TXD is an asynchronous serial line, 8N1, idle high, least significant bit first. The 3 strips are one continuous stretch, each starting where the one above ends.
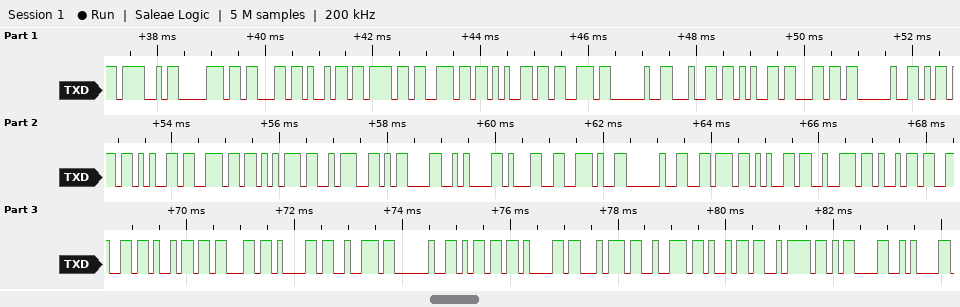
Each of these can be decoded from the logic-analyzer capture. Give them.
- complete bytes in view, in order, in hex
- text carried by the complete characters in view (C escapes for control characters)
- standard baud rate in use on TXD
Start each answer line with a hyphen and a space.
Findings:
- 4F 70 63 69 6F 6E 65 73 20 64 65 6C 20 6D 65 6E 75 3A 0D 0A 31 2E 20 76 65 72 69 66 69 63 61 72 20 6D 61 74 72 69 7A 0D 0A
- "Opciones del menu:\r\n1. verificar matriz\r\n"
- 9600 baud
